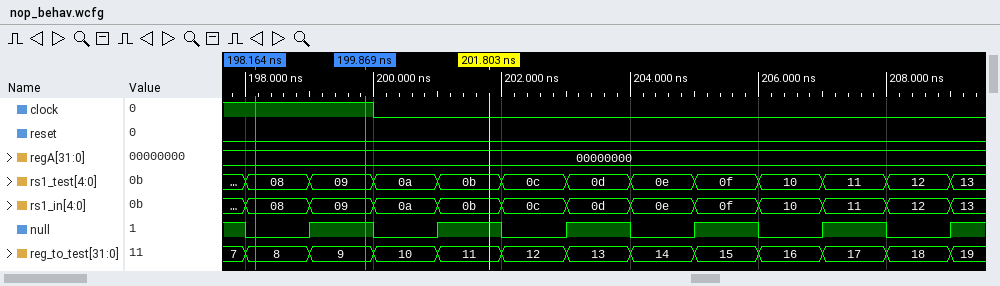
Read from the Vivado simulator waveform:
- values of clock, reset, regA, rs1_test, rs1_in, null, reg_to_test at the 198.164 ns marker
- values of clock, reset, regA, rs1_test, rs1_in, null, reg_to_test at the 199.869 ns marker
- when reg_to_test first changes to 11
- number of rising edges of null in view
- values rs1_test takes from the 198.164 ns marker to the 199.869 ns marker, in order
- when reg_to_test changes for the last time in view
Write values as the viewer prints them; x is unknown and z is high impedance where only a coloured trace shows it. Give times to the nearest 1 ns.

clock=1, reset=0, regA=00000000, rs1_test=08, rs1_in=08, null=0, reg_to_test=8
clock=1, reset=0, regA=00000000, rs1_test=09, rs1_in=09, null=1, reg_to_test=9
201 ns
6
08, 09
209 ns
